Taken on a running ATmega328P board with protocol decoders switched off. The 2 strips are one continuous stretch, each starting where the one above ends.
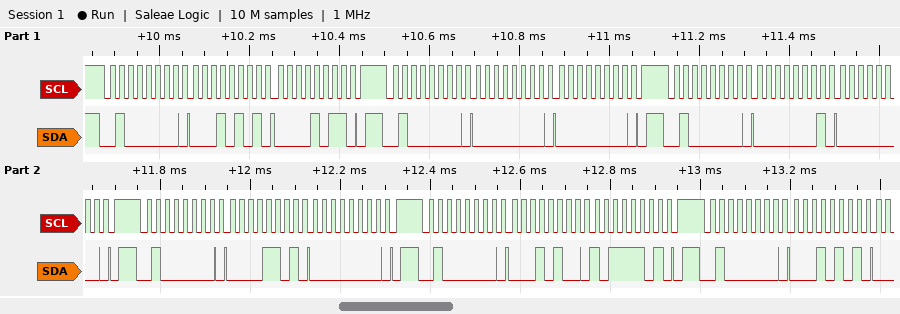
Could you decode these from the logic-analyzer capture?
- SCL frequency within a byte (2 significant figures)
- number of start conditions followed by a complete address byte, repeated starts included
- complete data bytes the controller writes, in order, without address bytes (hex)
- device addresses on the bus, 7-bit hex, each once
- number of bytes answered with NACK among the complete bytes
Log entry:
50 kHz
6
15 0B 00 00 01 00 0D 00 14 BD 15
0x20
0
